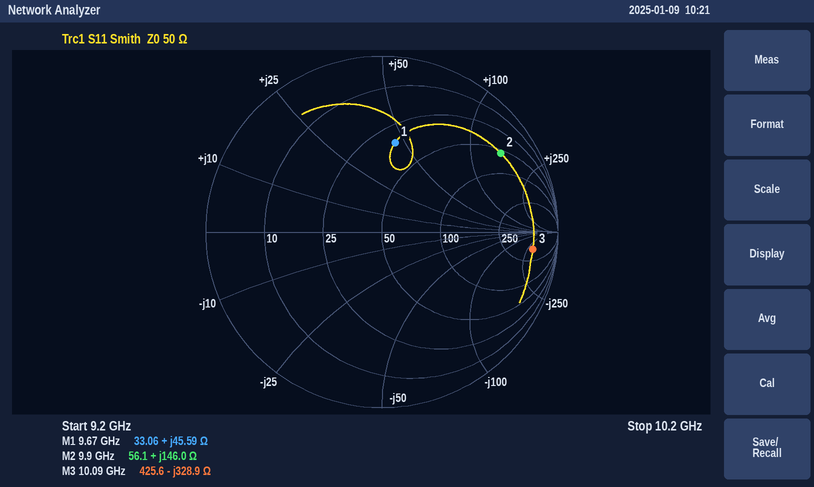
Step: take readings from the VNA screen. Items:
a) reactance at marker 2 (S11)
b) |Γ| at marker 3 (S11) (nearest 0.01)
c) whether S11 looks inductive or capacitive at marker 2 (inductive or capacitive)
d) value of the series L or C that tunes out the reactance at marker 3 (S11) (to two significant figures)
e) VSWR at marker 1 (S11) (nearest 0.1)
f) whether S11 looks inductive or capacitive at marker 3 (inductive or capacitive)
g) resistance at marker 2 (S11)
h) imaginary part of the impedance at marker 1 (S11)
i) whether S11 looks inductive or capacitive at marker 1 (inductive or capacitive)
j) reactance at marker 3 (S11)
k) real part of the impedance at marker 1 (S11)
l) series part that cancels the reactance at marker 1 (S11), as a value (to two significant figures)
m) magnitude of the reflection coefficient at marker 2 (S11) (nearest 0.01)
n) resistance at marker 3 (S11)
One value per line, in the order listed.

+146.0 Ω
0.86
inductive
5.2 nH
3.1
capacitive
56.1 Ω
+45.59 Ω
inductive
-328.9 Ω
33.06 Ω
360 fF
0.81
425.6 Ω
